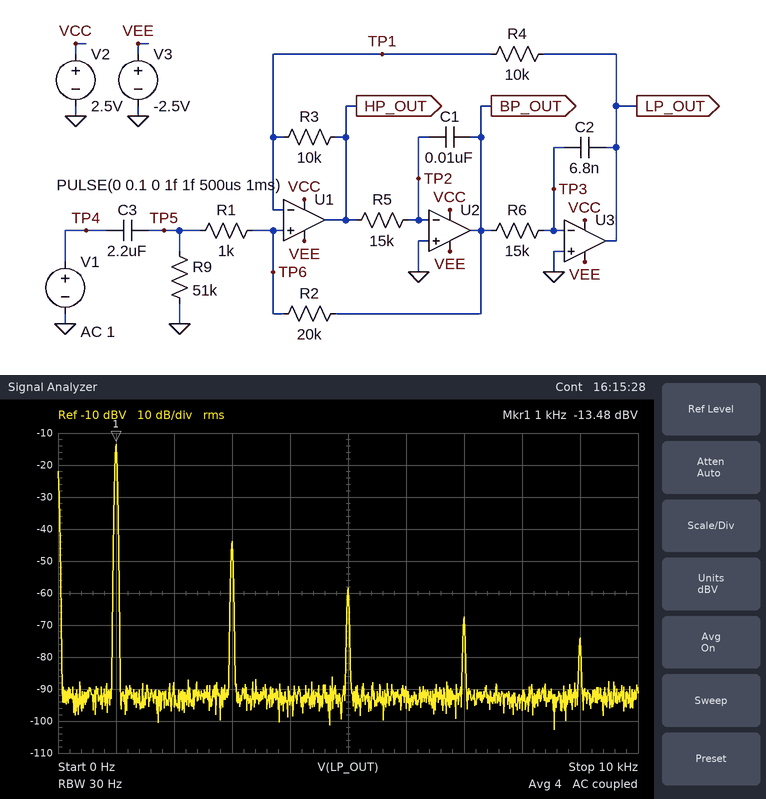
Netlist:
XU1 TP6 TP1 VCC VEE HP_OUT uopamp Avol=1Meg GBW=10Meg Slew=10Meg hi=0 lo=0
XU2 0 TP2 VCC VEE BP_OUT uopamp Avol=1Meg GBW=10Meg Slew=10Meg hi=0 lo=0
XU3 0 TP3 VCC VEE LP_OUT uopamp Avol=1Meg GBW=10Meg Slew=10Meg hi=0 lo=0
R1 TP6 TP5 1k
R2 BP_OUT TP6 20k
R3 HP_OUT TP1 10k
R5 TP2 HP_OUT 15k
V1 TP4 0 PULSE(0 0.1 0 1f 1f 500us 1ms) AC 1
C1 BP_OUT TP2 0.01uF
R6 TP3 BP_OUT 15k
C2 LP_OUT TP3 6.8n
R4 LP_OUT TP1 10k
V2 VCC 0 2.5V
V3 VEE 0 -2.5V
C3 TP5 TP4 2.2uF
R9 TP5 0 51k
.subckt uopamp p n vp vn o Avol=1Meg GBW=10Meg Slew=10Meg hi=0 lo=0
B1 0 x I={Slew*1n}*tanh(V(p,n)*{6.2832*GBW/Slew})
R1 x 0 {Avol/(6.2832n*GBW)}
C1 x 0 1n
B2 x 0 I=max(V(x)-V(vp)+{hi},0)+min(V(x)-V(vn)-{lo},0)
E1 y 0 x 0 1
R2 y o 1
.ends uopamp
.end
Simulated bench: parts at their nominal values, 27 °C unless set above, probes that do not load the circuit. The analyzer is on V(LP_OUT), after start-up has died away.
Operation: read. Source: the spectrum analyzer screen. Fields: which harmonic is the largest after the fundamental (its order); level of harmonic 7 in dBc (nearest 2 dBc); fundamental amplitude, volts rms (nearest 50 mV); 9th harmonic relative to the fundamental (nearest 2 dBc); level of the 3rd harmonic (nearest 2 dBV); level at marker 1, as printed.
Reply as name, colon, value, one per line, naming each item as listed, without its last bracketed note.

which harmonic is the largest after the fundamental: 3
level of harmonic 7 in dBc: -54 dBc
fundamental amplitude, volts rms: 200 mV
9th harmonic relative to the fundamental: -60 dBc
level of the 3rd harmonic: -44 dBV
level at marker 1, as printed: -13.48 dBV
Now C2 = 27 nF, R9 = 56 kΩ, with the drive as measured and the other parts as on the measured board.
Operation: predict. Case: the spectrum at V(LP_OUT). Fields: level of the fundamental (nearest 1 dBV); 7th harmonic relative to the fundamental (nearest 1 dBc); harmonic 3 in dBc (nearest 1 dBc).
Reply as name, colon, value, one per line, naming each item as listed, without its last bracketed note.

level of the fundamental: -24 dBV
7th harmonic relative to the fundamental: -55 dBc
harmonic 3 in dBc: -33 dBc
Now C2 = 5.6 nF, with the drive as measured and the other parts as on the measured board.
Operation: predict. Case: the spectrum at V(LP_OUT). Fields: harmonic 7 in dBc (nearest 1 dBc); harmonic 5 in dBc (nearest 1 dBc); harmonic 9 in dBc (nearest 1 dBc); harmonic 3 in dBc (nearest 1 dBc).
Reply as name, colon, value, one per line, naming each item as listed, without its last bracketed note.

harmonic 7 in dBc: -50 dBc
harmonic 5 in dBc: -41 dBc
harmonic 9 in dBc: -57 dBc
harmonic 3 in dBc: -26 dBc
